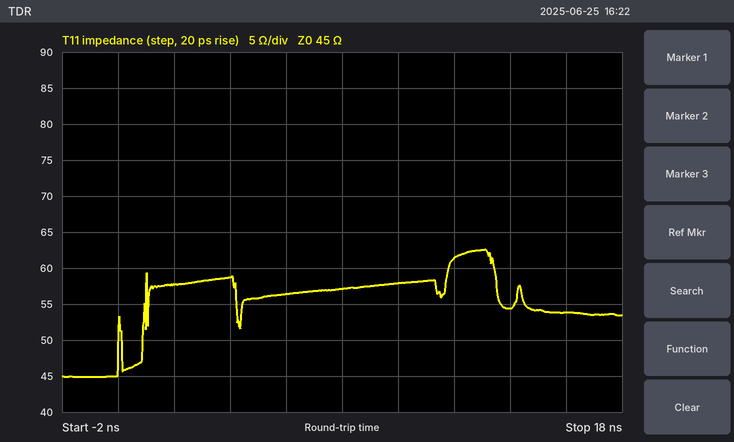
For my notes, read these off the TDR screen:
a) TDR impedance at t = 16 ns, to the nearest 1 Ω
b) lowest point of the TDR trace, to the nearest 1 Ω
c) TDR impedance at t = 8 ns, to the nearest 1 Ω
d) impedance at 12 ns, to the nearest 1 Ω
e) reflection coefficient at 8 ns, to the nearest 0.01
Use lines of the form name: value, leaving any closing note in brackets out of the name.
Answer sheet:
TDR impedance at t = 16 ns, to the nearest 1 Ω: 54 Ω
lowest point of the TDR trace, to the nearest 1 Ω: 45 Ω
TDR impedance at t = 8 ns, to the nearest 1 Ω: 57 Ω
impedance at 12 ns, to the nearest 1 Ω: 61 Ω
reflection coefficient at 8 ns, to the nearest 0.01: +0.12
